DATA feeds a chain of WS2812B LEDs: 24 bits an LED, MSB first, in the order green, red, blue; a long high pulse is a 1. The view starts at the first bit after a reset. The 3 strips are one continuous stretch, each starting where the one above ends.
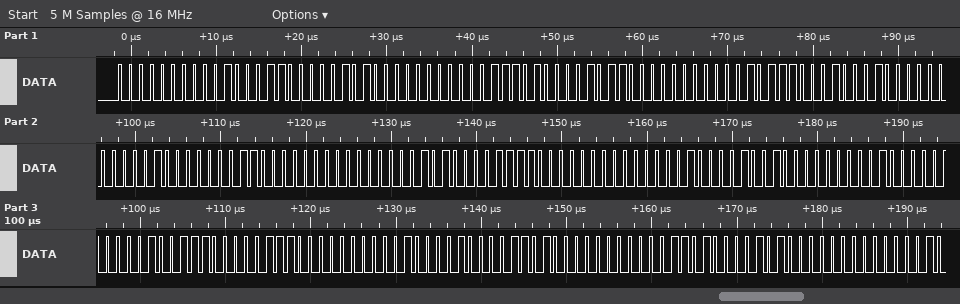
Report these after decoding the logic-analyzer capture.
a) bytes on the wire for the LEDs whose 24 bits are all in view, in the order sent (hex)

00 23 05 00 1D 0B 00 17 11 00 10 18 00 0A 1E 00 04 24 01 00 27 07 00 21 0D 00 1A
